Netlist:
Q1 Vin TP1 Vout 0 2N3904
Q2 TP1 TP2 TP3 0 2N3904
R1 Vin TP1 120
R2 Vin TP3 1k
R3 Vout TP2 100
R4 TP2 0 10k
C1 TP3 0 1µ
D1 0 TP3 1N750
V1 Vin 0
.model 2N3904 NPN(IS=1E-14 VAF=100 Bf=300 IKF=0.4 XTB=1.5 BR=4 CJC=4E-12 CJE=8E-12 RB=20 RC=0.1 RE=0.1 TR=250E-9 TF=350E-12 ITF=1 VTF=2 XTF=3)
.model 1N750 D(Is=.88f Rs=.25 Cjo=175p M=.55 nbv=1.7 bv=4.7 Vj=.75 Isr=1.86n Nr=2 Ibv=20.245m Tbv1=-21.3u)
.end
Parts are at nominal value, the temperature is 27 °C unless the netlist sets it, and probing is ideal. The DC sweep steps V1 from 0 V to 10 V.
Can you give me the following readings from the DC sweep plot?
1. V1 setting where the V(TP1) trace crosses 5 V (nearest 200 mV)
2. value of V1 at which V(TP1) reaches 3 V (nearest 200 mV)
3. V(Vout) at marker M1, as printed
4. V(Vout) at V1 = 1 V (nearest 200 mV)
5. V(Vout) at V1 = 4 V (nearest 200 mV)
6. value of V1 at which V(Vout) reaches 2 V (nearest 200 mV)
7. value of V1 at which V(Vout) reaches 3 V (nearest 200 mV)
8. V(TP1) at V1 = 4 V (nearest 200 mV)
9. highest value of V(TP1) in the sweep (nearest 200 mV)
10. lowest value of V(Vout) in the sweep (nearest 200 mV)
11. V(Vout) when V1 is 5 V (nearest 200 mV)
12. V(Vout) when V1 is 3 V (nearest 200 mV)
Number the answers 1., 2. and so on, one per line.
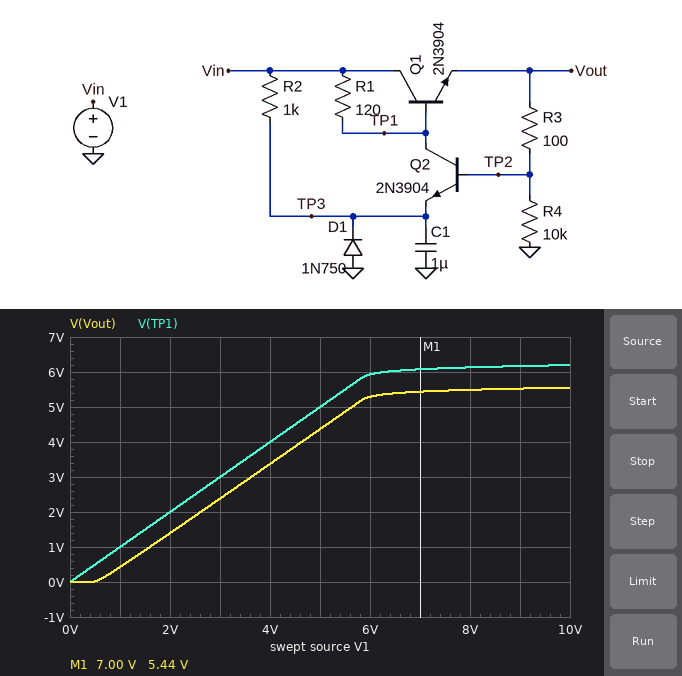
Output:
1. 5.0 V
2. 3.0 V
3. 5.44 V
4. 400 mV
5. 3.4 V
6. 2.6 V
7. 3.6 V
8. 4.0 V
9. 6.2 V
10. 0 V
11. 4.4 V
12. 2.4 V
